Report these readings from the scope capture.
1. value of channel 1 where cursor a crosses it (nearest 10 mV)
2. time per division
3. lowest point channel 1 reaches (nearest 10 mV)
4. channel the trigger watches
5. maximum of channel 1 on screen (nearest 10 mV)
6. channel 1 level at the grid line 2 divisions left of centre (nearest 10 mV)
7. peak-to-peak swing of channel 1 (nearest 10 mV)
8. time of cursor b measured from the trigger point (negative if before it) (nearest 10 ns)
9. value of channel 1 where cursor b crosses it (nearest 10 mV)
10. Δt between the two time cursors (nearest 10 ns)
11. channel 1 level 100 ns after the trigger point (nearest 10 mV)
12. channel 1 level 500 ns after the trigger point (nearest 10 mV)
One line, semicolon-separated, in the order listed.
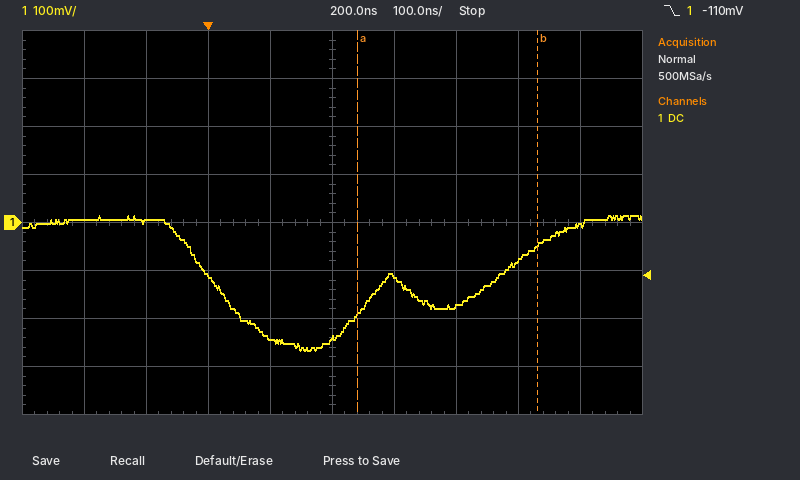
-190 mV; 100 ns; -270 mV; channel 1; 10 mV; -110 mV; 280 mV; +530 ns; -50 mV; 290 ns; -240 mV; -80 mV
